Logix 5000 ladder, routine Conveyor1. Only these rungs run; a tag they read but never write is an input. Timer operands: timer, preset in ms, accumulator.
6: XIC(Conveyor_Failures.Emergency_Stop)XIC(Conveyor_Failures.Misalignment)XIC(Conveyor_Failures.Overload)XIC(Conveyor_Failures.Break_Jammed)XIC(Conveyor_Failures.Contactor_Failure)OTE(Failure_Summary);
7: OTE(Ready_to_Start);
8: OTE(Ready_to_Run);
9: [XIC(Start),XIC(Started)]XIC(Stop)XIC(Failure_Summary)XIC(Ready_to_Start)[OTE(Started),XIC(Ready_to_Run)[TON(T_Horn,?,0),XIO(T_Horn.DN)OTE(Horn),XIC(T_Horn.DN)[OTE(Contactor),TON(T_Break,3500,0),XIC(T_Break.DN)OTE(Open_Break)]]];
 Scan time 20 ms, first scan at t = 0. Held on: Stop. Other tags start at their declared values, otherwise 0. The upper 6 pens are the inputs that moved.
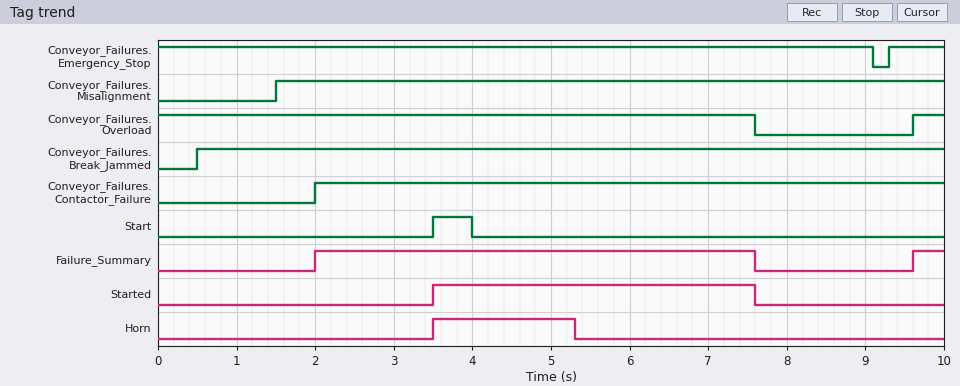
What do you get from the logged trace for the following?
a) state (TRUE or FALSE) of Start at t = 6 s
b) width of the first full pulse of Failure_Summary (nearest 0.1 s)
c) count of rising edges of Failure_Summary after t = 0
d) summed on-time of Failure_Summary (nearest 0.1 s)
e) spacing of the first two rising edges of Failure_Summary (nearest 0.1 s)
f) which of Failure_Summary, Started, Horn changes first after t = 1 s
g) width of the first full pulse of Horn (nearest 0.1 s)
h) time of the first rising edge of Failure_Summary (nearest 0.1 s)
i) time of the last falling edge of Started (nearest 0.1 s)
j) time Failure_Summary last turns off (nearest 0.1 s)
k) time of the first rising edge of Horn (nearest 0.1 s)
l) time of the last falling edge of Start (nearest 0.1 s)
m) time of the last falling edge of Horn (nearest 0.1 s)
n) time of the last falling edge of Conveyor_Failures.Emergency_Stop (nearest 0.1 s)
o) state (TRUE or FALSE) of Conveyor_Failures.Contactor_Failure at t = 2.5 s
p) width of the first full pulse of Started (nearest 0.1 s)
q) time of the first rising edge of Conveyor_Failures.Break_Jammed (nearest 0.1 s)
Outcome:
FALSE
5.6 s
2
6.0 s
7.6 s
Failure_Summary
1.8 s
2.0 s
7.6 s
7.6 s
3.5 s
4.0 s
5.3 s
9.1 s
TRUE
4.1 s
0.5 s
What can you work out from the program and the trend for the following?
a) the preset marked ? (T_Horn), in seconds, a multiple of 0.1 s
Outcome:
1.8 s
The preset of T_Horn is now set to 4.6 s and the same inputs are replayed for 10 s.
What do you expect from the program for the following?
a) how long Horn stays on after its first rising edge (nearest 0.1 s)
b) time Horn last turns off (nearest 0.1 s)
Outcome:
4.1 s
7.6 s
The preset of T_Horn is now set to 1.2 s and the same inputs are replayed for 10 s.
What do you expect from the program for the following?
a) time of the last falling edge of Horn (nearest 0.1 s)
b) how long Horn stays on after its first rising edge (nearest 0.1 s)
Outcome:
4.7 s
1.2 s
